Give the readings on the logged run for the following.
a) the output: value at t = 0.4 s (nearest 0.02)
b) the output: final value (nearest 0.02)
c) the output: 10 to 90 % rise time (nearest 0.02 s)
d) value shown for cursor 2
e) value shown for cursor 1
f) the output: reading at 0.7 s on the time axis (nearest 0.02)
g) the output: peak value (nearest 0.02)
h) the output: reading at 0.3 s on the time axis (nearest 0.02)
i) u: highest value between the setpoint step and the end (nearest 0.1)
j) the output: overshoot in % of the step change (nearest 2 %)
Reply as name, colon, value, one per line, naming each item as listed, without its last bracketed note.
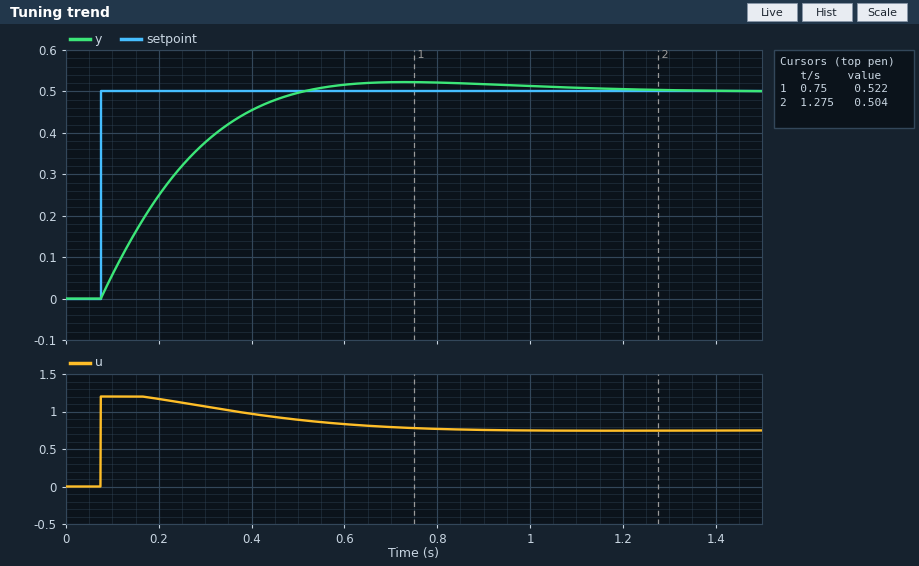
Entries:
the output: value at t = 0.4 s: 0.46
the output: final value: 0.50
the output: 10 to 90 % rise time: 0.30 s
value shown for cursor 2: 0.504
value shown for cursor 1: 0.522
the output: reading at 0.7 s on the time axis: 0.52
the output: peak value: 0.52
the output: reading at 0.3 s on the time axis: 0.38
u: highest value between the setpoint step and the end: 1.2
the output: overshoot in % of the step change: 4 %
